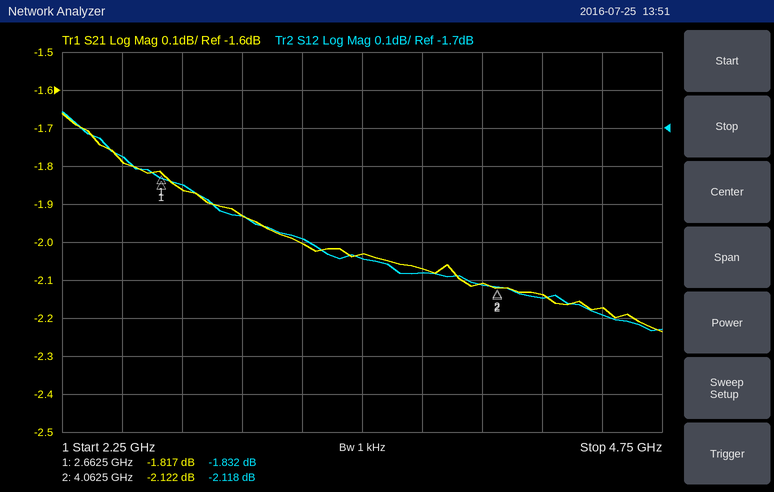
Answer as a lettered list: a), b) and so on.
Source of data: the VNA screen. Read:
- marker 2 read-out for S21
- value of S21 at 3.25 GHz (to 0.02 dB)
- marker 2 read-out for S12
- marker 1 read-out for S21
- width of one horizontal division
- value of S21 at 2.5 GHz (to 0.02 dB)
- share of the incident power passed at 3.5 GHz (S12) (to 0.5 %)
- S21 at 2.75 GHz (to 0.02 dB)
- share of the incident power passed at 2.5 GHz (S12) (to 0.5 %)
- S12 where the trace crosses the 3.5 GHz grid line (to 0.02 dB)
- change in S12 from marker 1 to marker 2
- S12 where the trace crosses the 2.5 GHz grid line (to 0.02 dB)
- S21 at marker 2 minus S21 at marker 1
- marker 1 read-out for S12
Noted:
a) -2.122 dB
b) -2.00 dB
c) -2.118 dB
d) -1.817 dB
e) 250 MHz
f) -1.78 dB
g) 62.5 %
h) -1.86 dB
i) 66.5 %
j) -2.04 dB
k) -0.286 dB
l) -1.78 dB
m) -0.305 dB
n) -1.832 dB
